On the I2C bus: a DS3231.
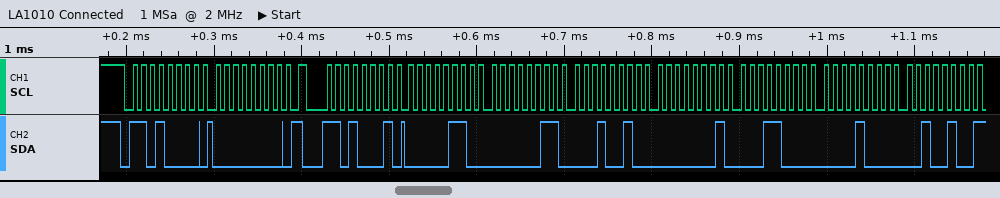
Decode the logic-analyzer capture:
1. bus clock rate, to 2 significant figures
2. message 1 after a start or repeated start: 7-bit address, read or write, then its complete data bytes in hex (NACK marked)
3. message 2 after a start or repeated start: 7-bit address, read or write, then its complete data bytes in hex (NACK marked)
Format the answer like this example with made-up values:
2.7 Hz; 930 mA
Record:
100 kHz; 0x68 write: 00; 0x68 read: 06 03 12 01 18 08 24 NACK
